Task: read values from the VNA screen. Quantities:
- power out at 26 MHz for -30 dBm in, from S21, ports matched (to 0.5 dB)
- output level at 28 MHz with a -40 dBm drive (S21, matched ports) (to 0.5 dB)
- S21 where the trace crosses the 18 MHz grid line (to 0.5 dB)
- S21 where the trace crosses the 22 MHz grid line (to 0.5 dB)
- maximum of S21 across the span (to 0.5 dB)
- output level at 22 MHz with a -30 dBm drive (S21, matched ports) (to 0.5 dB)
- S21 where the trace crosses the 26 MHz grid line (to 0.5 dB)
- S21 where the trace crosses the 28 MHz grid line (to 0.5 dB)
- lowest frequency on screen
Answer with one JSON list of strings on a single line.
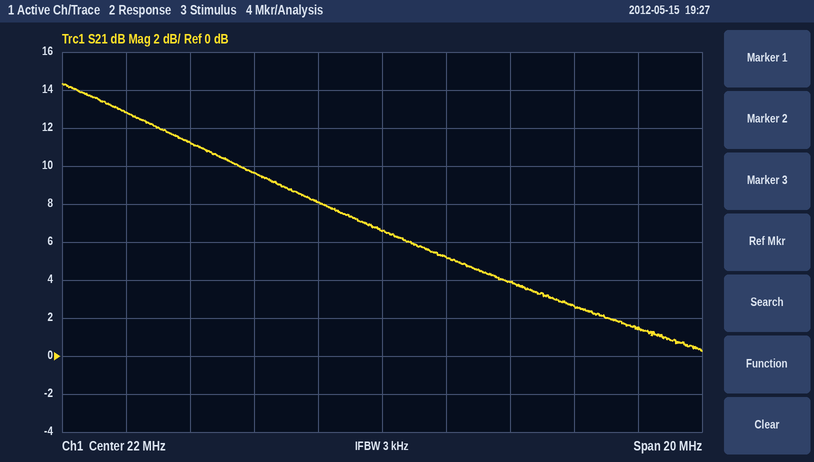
["-26.0 dBm", "-37.5 dBm", "9.5 dB", "6.5 dB", "14.5 dB", "-23.5 dBm", "4.0 dB", "2.5 dB", "12 MHz"]
